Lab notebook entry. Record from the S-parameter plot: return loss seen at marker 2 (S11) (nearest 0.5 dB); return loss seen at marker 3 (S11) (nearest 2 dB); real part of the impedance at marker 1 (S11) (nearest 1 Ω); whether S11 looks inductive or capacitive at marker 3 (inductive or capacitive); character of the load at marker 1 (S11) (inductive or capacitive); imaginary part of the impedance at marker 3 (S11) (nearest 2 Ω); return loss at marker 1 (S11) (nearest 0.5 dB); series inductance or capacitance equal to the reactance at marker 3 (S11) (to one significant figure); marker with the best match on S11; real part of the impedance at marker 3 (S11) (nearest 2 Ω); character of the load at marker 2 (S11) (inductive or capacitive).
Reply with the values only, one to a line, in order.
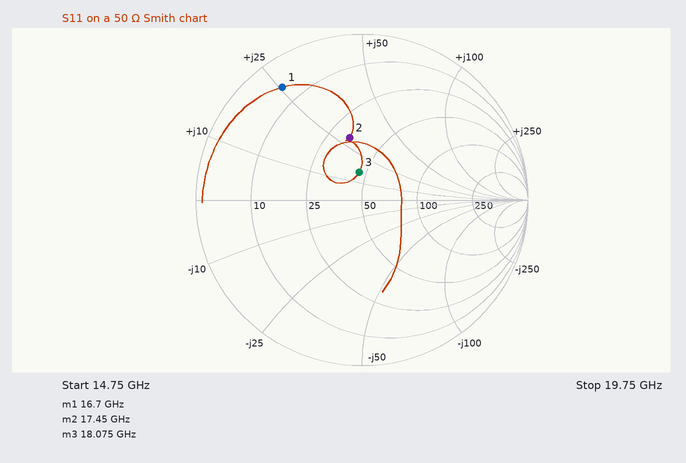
8.5 dB
16 dB
6 Ω
inductive
inductive
+16 Ω
1.5 dB
100 pH
marker 3
46 Ω
inductive
